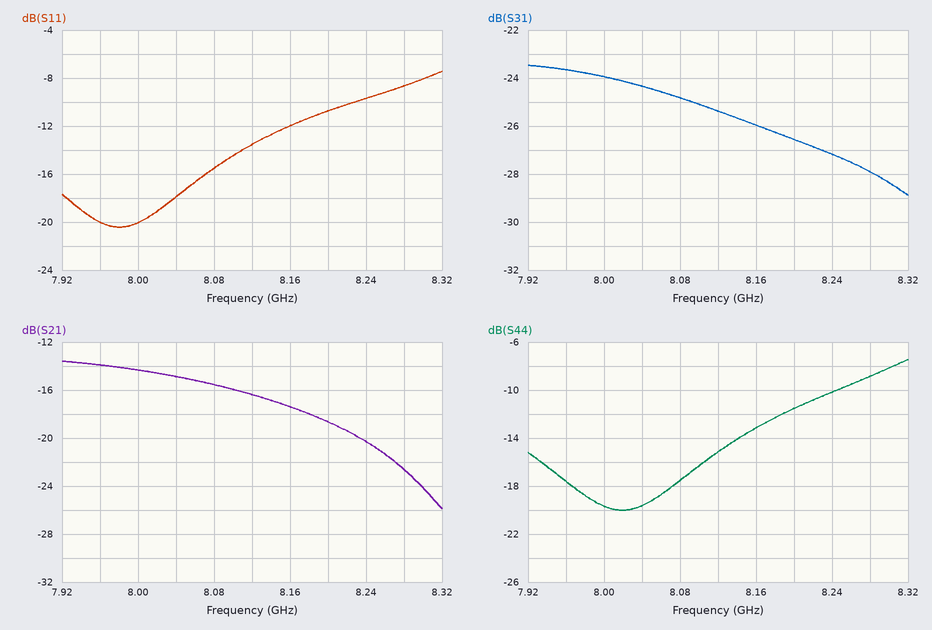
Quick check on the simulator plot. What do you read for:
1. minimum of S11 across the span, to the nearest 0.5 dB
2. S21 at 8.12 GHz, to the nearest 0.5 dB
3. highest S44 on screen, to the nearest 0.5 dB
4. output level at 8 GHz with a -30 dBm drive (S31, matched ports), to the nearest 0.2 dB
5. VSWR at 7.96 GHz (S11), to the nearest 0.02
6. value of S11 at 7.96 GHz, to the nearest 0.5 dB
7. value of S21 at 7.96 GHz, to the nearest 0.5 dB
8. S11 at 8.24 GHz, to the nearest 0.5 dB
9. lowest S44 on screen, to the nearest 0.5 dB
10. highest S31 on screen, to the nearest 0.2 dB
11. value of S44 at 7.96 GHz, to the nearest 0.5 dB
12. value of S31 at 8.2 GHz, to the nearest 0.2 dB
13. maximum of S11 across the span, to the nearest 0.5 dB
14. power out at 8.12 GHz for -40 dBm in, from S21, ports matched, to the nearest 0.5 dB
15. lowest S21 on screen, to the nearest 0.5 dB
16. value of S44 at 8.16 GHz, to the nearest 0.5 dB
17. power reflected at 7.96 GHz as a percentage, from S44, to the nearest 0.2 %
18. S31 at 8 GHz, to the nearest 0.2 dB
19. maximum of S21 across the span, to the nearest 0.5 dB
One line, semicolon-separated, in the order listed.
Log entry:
-20.5 dB; -16.5 dB; -7.5 dB; -54.0 dBm; 1.22; -20.0 dB; -14.0 dB; -9.5 dB; -20.0 dB; -23.4 dB; -17.5 dB; -26.6 dB; -7.5 dB; -56.5 dBm; -26.0 dB; -13.0 dB; 1.8 %; -24.0 dB; -13.5 dB
